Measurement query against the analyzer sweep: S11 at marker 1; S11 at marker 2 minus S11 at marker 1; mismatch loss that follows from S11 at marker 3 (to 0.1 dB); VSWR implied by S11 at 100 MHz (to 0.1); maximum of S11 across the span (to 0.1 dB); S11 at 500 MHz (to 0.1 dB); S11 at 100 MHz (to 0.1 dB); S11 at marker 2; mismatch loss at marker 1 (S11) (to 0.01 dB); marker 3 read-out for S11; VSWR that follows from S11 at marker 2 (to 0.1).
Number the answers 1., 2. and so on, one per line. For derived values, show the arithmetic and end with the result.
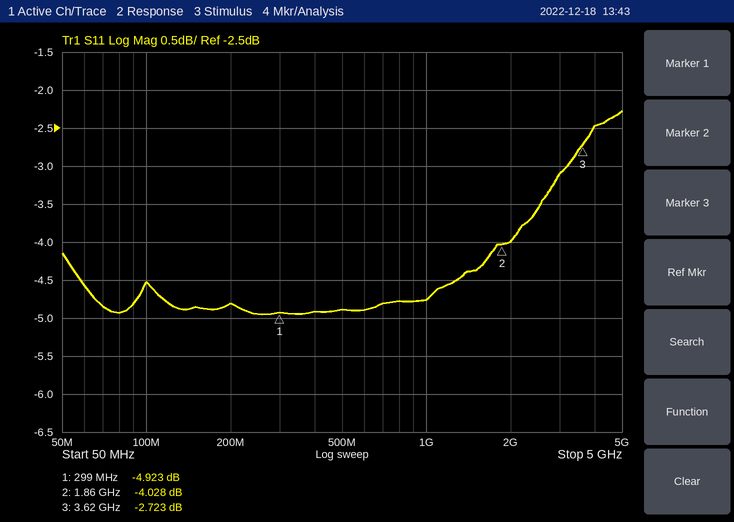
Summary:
1. -4.923 dB
2. -4.028 − (-4.923) = 0.895 dB
3. −10 log10(1 − 10^(-2.723/10)) ≈ 3.3 dB
4. |Γ| = 10^(-4.5/20) = 0.5957; VSWR = (1 + 0.5957)/(1 − 0.5957) ≈ 3.9
5. -2.3 dB
6. -4.9 dB
7. -4.5 dB
8. -4.028 dB
9. −10 log10(1 − 10^(-4.923/10)) ≈ 1.69 dB
10. -2.723 dB
11. (1 + 0.6289)/(1 − 0.6289) ≈ 4.4
